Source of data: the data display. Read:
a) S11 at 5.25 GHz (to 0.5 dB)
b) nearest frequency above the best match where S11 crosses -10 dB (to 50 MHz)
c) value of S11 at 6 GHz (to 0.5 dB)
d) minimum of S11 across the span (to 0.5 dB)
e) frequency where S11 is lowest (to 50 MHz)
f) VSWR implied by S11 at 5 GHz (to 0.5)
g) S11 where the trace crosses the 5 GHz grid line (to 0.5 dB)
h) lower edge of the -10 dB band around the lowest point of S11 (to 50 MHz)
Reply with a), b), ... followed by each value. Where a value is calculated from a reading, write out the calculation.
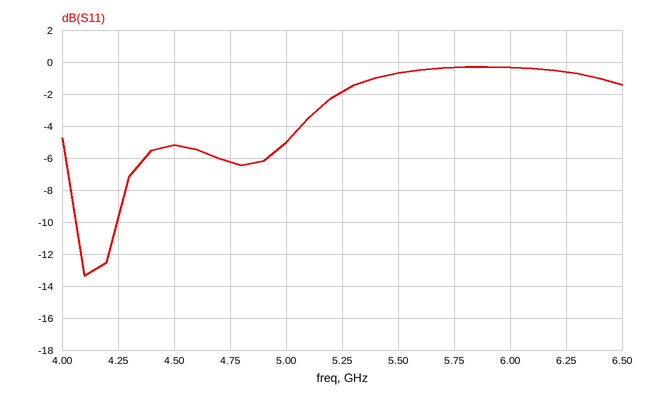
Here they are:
a) -2.0 dB
b) 4.25 GHz
c) -0.5 dB
d) -13.5 dB
e) 4.10 GHz
f) |Γ| = 10^(-5/20) = 0.5623; VSWR = (1 + 0.5623)/(1 − 0.5623) ≈ 3.57, so 3.5 to the nearest 0.5
g) -5.0 dB
h) 4.05 GHz
